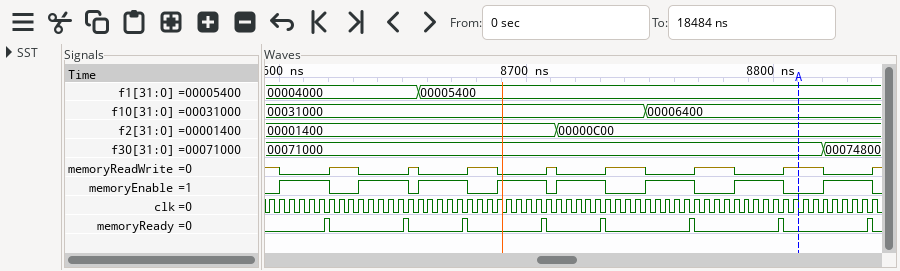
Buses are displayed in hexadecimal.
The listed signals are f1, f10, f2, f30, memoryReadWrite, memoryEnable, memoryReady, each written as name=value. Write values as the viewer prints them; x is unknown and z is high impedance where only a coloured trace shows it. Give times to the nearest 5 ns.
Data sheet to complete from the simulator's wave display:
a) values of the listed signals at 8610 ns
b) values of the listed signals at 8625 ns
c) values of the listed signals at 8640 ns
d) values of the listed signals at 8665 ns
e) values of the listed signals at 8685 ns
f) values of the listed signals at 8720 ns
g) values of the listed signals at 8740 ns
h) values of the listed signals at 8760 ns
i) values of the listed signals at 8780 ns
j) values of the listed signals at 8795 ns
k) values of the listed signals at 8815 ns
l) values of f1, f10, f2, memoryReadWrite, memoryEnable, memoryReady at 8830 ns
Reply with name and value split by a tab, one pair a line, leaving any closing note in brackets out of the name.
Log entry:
values of the listed signals at 8610 ns	f1=00004000, f10=00031000, f2=00001400, f30=00071000, memoryReadWrite=0, memoryEnable=1, memoryReady=0
values of the listed signals at 8625 ns	f1=00004000, f10=00031000, f2=00001400, f30=00071000, memoryReadWrite=z, memoryEnable=0, memoryReady=0
values of the listed signals at 8640 ns	f1=00004000, f10=00031000, f2=00001400, f30=00071000, memoryReadWrite=0, memoryEnable=1, memoryReady=0
values of the listed signals at 8665 ns	f1=00005400, f10=00031000, f2=00001400, f30=00071000, memoryReadWrite=0, memoryEnable=1, memoryReady=0
values of the listed signals at 8685 ns	f1=00005400, f10=00031000, f2=00001400, f30=00071000, memoryReadWrite=z, memoryEnable=0, memoryReady=0
values of the listed signals at 8720 ns	f1=00005400, f10=00031000, f2=00000C00, f30=00071000, memoryReadWrite=0, memoryEnable=1, memoryReady=0
values of the listed signals at 8740 ns	f1=00005400, f10=00031000, f2=00000C00, f30=00071000, memoryReadWrite=z, memoryEnable=0, memoryReady=0
values of the listed signals at 8760 ns	f1=00005400, f10=00006400, f2=00000C00, f30=00071000, memoryReadWrite=0, memoryEnable=1, memoryReady=0
values of the listed signals at 8780 ns	f1=00005400, f10=00006400, f2=00000C00, f30=00071000, memoryReadWrite=z, memoryEnable=0, memoryReady=0
values of the listed signals at 8795 ns	f1=00005400, f10=00006400, f2=00000C00, f30=00071000, memoryReadWrite=0, memoryEnable=1, memoryReady=0
values of the listed signals at 8815 ns	f1=00005400, f10=00006400, f2=00000C00, f30=00071000, memoryReadWrite=z, memoryEnable=0, memoryReady=0
values of f1, f10, f2, memoryReadWrite, memoryEnable, memoryReady at 8830 ns	f1=00005400, f10=00006400, f2=00000C00, memoryReadWrite=0, memoryEnable=1, memoryReady=0
